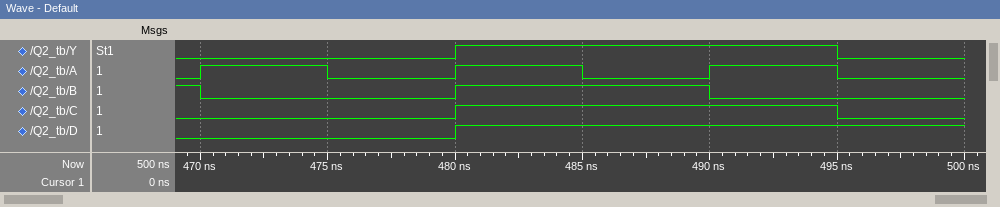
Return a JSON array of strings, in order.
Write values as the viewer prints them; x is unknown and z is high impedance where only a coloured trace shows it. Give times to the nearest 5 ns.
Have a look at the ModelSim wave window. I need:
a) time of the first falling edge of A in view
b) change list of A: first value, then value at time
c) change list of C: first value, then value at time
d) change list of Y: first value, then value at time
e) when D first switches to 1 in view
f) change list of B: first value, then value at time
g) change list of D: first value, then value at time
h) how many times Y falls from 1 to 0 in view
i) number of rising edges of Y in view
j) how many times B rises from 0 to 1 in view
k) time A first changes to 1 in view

["475 ns", "0, 1 at 470 ns, 0 at 475 ns, 1 at 480 ns, 0 at 485 ns, 1 at 490 ns, 0 at 495 ns", "0, 1 at 480 ns, 0 at 495 ns", "0, 1 at 480 ns, 0 at 495 ns", "480 ns", "1, 0 at 470 ns, 1 at 480 ns, 0 at 490 ns", "0, 1 at 480 ns", "1", "1", "1", "470 ns"]
